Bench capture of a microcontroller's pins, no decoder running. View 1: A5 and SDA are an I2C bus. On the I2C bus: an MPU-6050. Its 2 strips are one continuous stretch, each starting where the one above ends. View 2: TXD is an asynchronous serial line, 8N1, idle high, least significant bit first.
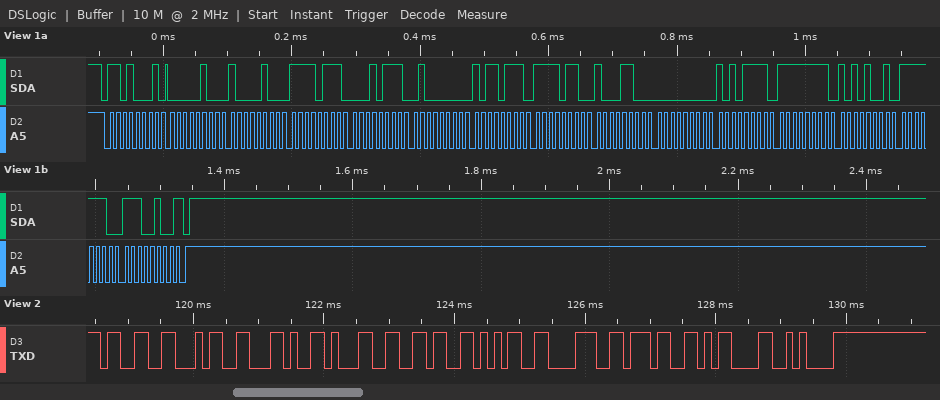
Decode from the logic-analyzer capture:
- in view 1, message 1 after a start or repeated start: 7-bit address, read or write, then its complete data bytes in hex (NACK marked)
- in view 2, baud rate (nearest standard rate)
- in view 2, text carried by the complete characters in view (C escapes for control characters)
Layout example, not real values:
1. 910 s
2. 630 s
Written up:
1. 0x68 read: 04 84 F7 17 40 B7 F6 8C 00 AF FF A9 FE E4 NACK
2. 9600 baud
3. "34,16587\r\n"
